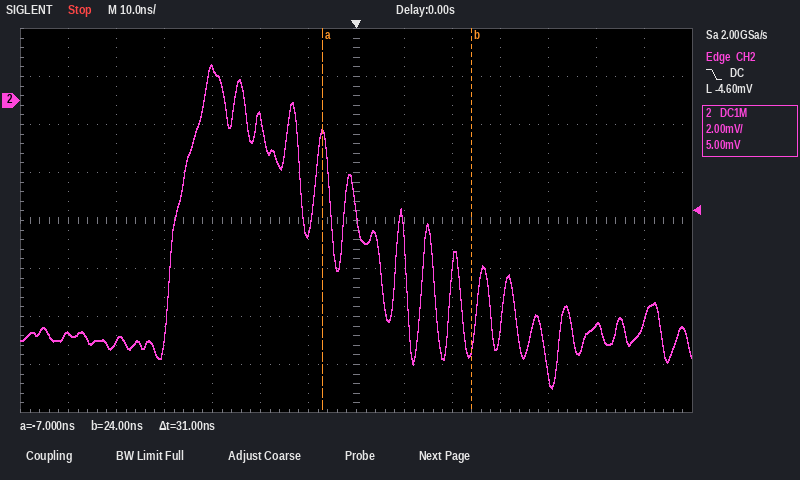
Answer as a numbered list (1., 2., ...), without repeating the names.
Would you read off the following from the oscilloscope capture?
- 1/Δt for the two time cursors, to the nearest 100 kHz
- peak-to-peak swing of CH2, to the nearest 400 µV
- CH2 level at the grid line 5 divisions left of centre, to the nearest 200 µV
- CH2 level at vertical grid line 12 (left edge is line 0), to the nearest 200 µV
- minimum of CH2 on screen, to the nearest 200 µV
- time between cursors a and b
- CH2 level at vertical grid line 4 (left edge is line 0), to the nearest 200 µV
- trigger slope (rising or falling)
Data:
1. 32.3 MHz
2. 13.6 mV
3. -10.0 mV
4. -9.4 mV
5. -12.0 mV
6. 31 ns
7. 1.4 mV
8. falling
